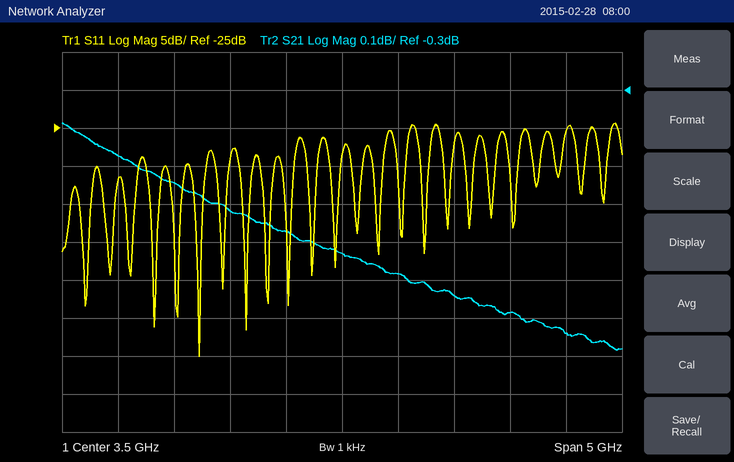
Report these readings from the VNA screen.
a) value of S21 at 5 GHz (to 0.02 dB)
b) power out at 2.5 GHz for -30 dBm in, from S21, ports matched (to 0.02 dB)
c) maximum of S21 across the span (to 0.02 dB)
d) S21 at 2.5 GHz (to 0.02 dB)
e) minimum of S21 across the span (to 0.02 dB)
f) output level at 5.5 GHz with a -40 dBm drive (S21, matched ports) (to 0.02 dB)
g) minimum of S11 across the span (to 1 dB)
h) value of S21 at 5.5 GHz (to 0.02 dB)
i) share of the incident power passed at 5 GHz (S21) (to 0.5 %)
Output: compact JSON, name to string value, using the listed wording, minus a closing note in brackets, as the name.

{"value of S21 at 5 GHz": "-0.88 dB", "power out at 2.5 GHz for -30 dBm in, from S21, ports matched": "-30.62 dBm", "maximum of S21 across the span": "-0.38 dB", "S21 at 2.5 GHz": "-0.62 dB", "minimum of S21 across the span": "-0.98 dB", "output level at 5.5 GHz with a -40 dBm drive (S21, matched ports)": "-40.94 dBm", "minimum of S11 across the span": "-55 dB", "value of S21 at 5.5 GHz": "-0.94 dB", "share of the incident power passed at 5 GHz (S21)": "81.5 %"}
